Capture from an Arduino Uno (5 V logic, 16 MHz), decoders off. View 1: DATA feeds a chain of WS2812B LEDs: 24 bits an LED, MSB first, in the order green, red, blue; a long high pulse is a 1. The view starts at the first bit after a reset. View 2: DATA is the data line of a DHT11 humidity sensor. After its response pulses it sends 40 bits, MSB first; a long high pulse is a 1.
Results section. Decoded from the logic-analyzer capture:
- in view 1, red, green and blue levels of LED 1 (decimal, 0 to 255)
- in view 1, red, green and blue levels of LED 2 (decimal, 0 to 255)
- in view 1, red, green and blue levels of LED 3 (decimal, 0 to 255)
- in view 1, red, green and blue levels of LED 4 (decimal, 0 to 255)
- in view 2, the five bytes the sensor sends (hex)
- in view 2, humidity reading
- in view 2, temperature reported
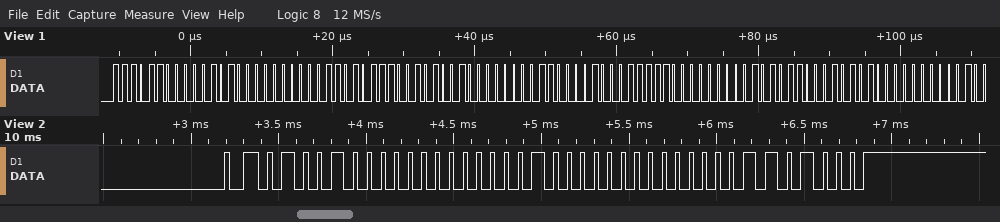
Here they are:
20, 236, 0
41, 215, 0
62, 194, 0
84, 172, 0
48 00 20 00 68
72 %
32.0 °C
